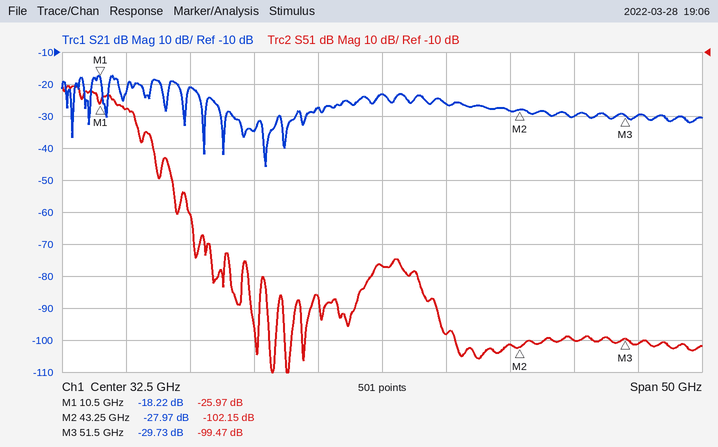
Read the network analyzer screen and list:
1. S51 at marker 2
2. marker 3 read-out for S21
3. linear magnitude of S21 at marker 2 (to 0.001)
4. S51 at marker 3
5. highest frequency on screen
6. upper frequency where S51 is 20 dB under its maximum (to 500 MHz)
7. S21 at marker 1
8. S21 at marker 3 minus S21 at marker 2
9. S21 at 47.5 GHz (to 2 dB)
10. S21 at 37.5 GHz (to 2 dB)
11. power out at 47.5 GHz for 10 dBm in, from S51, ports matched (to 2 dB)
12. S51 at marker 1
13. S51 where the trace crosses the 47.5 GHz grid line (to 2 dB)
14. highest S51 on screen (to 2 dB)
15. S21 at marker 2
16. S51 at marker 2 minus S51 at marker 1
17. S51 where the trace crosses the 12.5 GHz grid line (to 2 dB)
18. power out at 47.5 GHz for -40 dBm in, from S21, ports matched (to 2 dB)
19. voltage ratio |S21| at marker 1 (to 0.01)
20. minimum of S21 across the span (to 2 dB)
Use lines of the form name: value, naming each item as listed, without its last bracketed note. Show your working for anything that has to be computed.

S51 at marker 2: -102.15 dB
marker 3 read-out for S21: -29.73 dB
linear magnitude of S21 at marker 2: 10^(-27.97/20) ≈ 0.040
S51 at marker 3: -99.47 dB
highest frequency on screen: 57.5 GHz
upper frequency where S51 is 20 dB under its maximum: 14.5 GHz
S21 at marker 1: -18.22 dB
S21 at marker 3 minus S21 at marker 2: -29.73 − (-27.97) = -1.76 dB
S21 at 47.5 GHz: -30 dB
S21 at 37.5 GHz: -26 dB
power out at 47.5 GHz for 10 dBm in, from S51, ports matched: 10 dBm + (-100 dB) = -90 dBm
S51 at marker 1: -25.97 dB
S51 where the trace crosses the 47.5 GHz grid line: -100 dB
highest S51 on screen: -20 dB
S21 at marker 2: -27.97 dB
S51 at marker 2 minus S51 at marker 1: -102.15 − (-25.97) = -76.18 dB
S51 where the trace crosses the 12.5 GHz grid line: -28 dB
power out at 47.5 GHz for -40 dBm in, from S21, ports matched: -40 dBm + (-30 dB) = -70 dBm
voltage ratio |S21| at marker 1: 10^(-18.22/20) ≈ 0.12
minimum of S21 across the span: -46 dB
